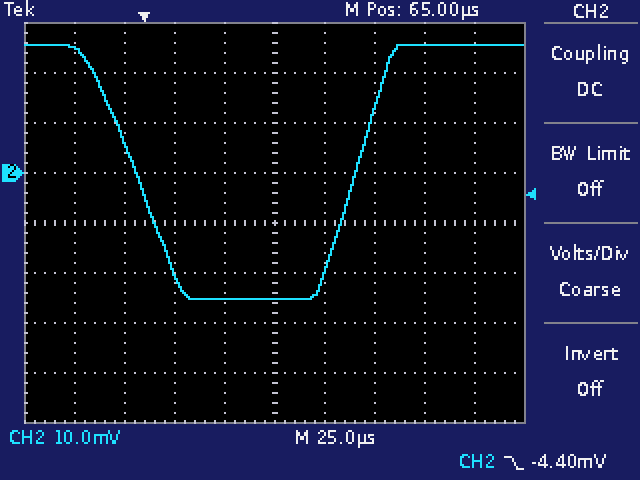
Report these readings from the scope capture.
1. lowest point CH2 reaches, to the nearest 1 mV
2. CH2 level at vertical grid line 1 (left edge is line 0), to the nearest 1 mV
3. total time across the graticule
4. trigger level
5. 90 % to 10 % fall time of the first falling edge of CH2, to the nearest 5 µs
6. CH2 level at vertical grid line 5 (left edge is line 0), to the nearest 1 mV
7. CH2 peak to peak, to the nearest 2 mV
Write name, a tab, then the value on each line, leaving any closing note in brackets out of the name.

lowest point CH2 reaches, to the nearest 1 mV	-25 mV
CH2 level at vertical grid line 1 (left edge is line 0), to the nearest 1 mV	25 mV
total time across the graticule	250 µs
trigger level	-4.40 mV
90 % to 10 % fall time of the first falling edge of CH2, to the nearest 5 µs	40 µs
CH2 level at vertical grid line 5 (left edge is line 0), to the nearest 1 mV	-25 mV
CH2 peak to peak, to the nearest 2 mV	50 mV
